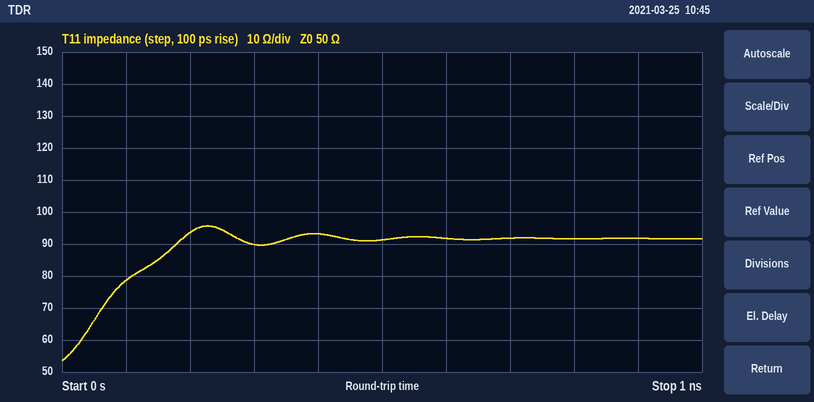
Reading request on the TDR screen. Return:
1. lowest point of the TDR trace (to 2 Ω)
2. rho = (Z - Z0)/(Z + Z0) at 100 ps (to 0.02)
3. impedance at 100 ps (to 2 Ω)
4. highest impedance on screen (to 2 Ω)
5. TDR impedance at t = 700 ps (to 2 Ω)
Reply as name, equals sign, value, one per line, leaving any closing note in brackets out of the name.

lowest point of the TDR trace = 54 Ω
rho = (Z - Z0)/(Z + Z0) at 100 ps = +0.22
impedance at 100 ps = 78 Ω
highest impedance on screen = 96 Ω
TDR impedance at t = 700 ps = 92 Ω
